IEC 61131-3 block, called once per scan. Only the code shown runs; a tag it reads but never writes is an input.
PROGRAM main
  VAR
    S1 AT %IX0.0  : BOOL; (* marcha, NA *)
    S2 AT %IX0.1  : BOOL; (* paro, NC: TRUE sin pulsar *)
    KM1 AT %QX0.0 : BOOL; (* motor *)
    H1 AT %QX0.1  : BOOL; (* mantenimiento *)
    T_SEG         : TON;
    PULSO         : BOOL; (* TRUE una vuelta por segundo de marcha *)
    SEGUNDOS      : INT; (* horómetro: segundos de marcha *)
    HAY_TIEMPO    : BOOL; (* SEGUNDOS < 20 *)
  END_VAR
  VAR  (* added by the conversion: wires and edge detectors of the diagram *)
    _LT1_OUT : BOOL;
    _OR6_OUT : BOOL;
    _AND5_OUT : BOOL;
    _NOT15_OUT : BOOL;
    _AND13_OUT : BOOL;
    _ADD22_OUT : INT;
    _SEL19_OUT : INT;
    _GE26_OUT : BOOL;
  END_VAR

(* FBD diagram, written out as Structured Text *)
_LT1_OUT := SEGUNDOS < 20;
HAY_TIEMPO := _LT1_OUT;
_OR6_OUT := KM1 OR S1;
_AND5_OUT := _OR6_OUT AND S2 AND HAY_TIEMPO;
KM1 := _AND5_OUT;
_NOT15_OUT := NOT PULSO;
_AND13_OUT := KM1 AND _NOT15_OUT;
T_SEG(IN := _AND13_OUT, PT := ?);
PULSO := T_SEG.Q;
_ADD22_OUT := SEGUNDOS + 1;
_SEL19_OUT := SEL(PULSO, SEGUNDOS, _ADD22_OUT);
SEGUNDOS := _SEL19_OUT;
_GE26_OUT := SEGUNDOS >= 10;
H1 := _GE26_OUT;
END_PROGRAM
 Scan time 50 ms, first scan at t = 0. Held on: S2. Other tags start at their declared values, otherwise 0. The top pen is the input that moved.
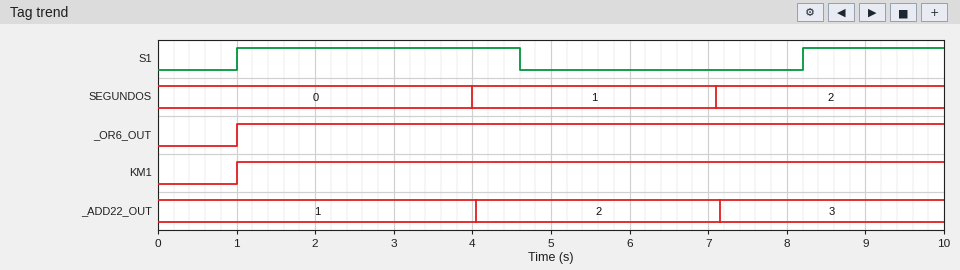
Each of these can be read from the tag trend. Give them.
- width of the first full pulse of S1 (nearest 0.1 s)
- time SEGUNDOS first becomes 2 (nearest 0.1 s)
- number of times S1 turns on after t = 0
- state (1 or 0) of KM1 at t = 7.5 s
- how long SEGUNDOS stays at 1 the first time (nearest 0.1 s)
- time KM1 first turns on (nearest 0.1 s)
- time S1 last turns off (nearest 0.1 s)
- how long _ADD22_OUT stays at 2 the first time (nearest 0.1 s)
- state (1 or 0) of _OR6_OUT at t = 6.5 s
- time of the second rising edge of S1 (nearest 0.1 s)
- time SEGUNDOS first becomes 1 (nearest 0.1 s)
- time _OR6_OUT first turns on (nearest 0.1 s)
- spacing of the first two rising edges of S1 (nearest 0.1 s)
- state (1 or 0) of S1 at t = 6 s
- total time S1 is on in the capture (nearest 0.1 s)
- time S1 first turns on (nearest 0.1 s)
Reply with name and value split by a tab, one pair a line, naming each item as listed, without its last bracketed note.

width of the first full pulse of S1	3.6 s
time SEGUNDOS first becomes 2	7.1 s
number of times S1 turns on after t = 0	2
state (1 or 0) of KM1 at t = 7.5 s	1
how long SEGUNDOS stays at 1 the first time	3.1 s
time KM1 first turns on	1.0 s
time S1 last turns off	4.6 s
how long _ADD22_OUT stays at 2 the first time	3.1 s
state (1 or 0) of _OR6_OUT at t = 6.5 s	1
time of the second rising edge of S1	8.2 s
time SEGUNDOS first becomes 1	4.0 s
time _OR6_OUT first turns on	1.0 s
spacing of the first two rising edges of S1	7.2 s
state (1 or 0) of S1 at t = 6 s	0
total time S1 is on in the capture	5.4 s
time S1 first turns on	1.0 s
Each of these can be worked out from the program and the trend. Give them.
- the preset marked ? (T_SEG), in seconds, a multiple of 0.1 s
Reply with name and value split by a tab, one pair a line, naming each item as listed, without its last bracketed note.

the preset marked ? (T_SEG), in seconds, a multiple of 0.1 s	3.0 s
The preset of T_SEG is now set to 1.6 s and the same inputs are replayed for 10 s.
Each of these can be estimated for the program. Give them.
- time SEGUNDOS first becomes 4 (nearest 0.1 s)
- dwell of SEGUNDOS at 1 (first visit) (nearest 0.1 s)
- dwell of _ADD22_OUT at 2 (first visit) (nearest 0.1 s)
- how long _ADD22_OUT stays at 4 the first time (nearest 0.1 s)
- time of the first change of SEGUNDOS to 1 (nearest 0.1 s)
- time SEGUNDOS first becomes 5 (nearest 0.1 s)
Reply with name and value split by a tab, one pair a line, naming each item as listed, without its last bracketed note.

time SEGUNDOS first becomes 4	7.7 s
dwell of SEGUNDOS at 1 (first visit)	1.7 s
dwell of _ADD22_OUT at 2 (first visit)	1.7 s
how long _ADD22_OUT stays at 4 the first time	1.7 s
time of the first change of SEGUNDOS to 1	2.6 s
time SEGUNDOS first becomes 5	9.4 s
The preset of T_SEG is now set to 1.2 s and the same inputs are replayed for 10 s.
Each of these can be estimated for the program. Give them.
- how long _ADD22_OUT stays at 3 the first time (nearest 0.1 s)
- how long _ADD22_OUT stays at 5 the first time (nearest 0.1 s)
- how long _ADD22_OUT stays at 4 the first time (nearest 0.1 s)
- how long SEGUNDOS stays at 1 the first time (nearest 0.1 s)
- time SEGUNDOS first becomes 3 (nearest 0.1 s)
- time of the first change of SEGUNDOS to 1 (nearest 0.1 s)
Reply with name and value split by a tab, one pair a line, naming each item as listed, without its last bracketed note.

how long _ADD22_OUT stays at 3 the first time	1.3 s
how long _ADD22_OUT stays at 5 the first time	1.3 s
how long _ADD22_OUT stays at 4 the first time	1.3 s
how long SEGUNDOS stays at 1 the first time	1.3 s
time SEGUNDOS first becomes 3	4.8 s
time of the first change of SEGUNDOS to 1	2.2 s
